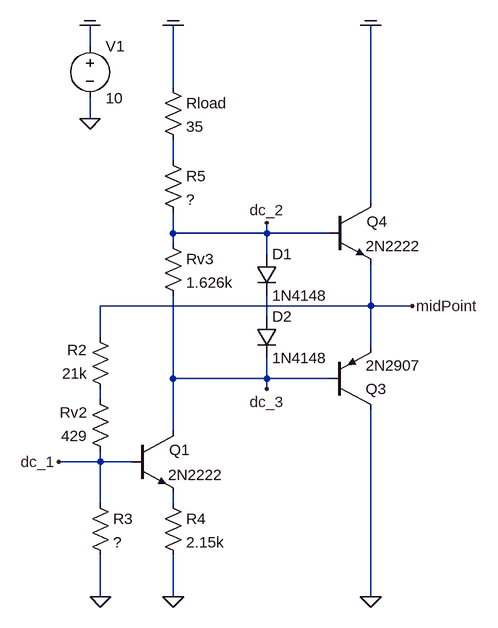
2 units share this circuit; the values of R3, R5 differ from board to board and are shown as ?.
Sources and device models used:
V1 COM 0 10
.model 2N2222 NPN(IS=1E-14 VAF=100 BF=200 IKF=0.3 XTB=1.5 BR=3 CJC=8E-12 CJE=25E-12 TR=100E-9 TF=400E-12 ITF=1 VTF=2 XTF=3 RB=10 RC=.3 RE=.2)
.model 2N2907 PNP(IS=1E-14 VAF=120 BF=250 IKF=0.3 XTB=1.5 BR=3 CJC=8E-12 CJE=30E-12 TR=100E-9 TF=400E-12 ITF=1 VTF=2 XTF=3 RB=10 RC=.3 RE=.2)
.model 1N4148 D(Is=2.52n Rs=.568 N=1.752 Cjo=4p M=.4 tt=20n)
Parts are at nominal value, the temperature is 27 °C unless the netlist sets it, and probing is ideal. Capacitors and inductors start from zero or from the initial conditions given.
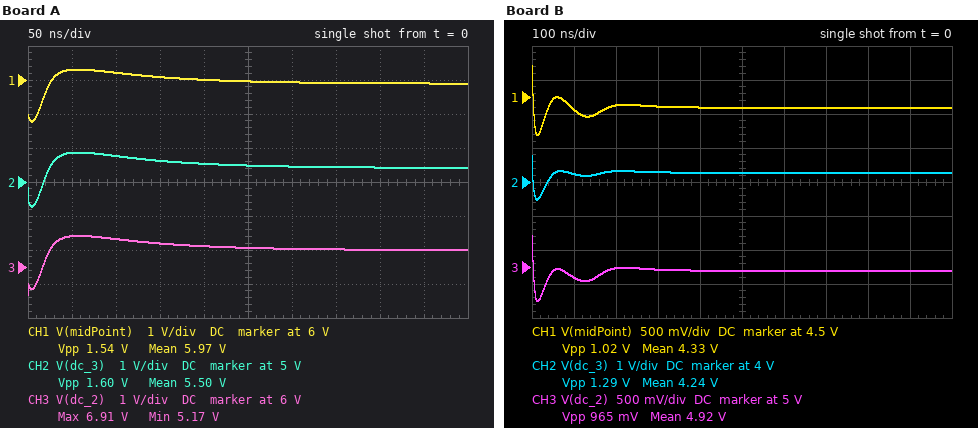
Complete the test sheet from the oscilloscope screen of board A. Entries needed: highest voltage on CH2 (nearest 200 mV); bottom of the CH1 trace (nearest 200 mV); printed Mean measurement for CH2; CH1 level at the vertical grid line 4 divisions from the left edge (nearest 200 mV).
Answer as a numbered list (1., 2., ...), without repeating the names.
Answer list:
1. 5.8 V
2. 4.8 V
3. 5.50 V
4. 6.0 V
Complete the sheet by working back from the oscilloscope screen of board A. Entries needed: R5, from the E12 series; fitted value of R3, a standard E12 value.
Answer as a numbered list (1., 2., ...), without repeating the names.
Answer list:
1. 3.3 kΩ
2. 22 kΩ
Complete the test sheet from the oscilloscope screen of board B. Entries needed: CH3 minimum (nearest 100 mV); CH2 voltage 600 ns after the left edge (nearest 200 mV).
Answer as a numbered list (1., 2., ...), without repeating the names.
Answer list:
1. 4.5 V
2. 4.2 V
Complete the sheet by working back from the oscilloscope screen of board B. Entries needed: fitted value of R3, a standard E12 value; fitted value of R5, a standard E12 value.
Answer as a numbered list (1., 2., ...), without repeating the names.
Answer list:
1. 12 kΩ
2. 12 kΩ
